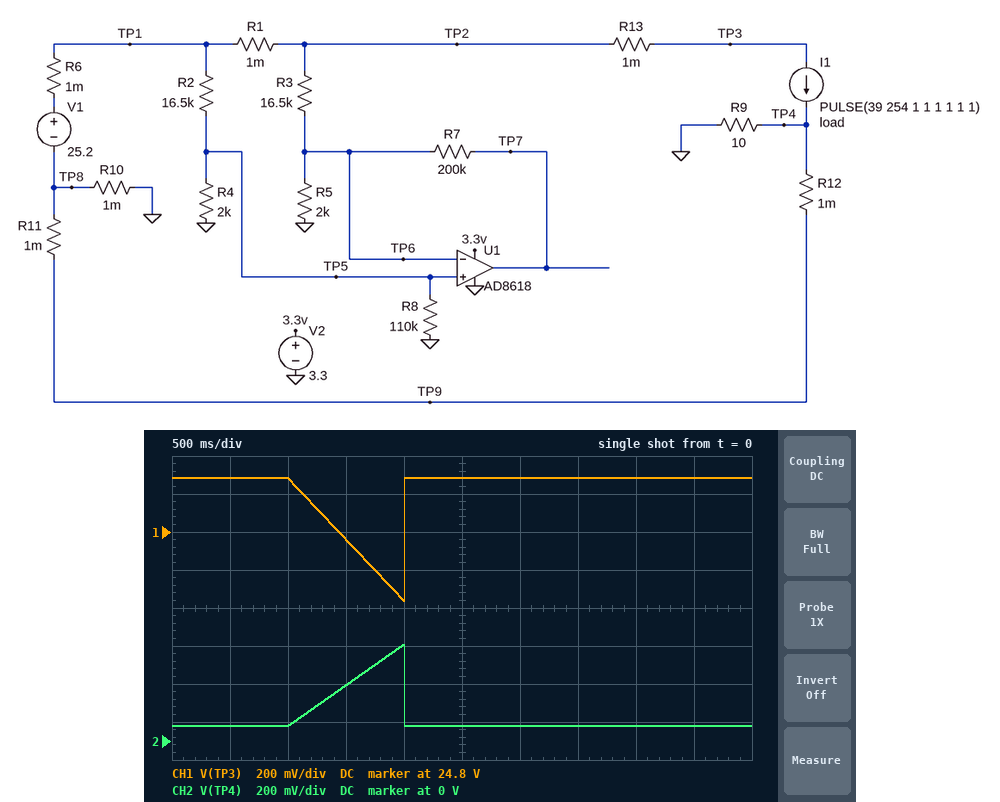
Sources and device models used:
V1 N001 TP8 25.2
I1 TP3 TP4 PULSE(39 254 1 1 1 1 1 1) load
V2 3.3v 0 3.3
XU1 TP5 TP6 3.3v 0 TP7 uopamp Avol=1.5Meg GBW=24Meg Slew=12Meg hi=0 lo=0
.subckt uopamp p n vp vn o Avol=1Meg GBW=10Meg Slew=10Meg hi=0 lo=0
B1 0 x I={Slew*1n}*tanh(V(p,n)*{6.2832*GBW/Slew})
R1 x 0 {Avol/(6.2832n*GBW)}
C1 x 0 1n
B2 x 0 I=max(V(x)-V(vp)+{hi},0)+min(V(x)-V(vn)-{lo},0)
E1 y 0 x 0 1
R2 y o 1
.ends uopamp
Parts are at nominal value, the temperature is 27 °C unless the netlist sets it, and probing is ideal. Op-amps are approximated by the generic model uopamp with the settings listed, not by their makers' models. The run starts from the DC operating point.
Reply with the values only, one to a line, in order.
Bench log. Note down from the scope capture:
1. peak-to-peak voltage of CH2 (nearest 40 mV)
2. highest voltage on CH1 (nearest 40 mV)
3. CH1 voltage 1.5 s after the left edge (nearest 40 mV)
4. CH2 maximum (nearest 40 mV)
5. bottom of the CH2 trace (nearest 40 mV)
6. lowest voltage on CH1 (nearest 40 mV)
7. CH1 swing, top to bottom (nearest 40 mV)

440 mV
25.08 V
24.76 V
520 mV
80 mV
24.44 V
640 mV
